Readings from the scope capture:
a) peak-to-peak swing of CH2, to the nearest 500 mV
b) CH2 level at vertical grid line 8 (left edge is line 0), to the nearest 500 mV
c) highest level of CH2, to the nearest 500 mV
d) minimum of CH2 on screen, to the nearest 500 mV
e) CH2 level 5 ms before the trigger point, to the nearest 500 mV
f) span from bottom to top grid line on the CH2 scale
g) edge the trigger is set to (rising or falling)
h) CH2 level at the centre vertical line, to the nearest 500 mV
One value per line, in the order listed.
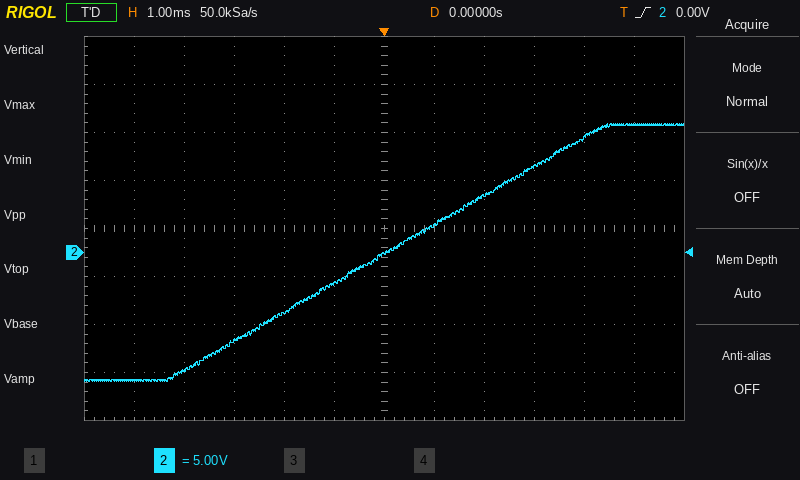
27.0 V
6.0 V
13.5 V
-13.5 V
-13.5 V
40 V
rising
0.0 V
